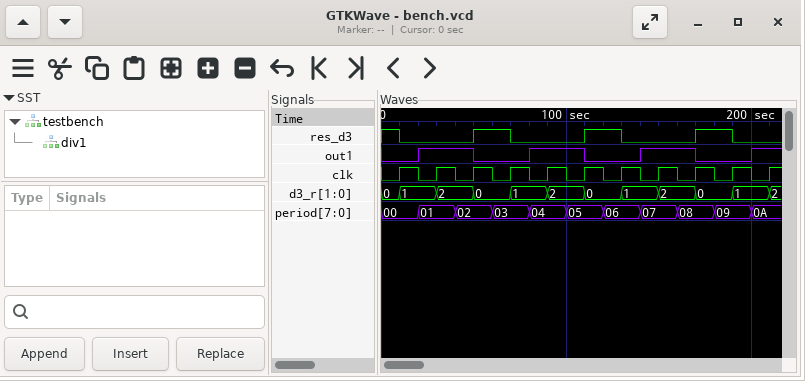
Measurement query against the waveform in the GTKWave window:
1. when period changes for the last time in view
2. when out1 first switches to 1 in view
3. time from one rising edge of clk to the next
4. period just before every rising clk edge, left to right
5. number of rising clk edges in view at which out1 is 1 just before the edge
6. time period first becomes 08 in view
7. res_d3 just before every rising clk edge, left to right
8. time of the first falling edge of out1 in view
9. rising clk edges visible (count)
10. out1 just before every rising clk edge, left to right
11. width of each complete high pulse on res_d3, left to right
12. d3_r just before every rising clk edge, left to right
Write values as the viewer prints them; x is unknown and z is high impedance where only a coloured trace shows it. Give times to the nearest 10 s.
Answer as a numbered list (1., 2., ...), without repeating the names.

1. 200 s
2. 20 s
3. 20 s
4. 00, 01, 02, 03, 04, 05, 06, 07, 08, 09, 0A
5. 7
6. 160 s
7. 1 0 0 1 0 0 1 0 0 1 0
8. 50 s
9. 11
10. 0 1 1 0 1 1 0 1 1 0 1
11. 20 s, 20 s, 20 s
12. 0, 1, 2, 0, 1, 2, 0, 1, 2, 0, 1
